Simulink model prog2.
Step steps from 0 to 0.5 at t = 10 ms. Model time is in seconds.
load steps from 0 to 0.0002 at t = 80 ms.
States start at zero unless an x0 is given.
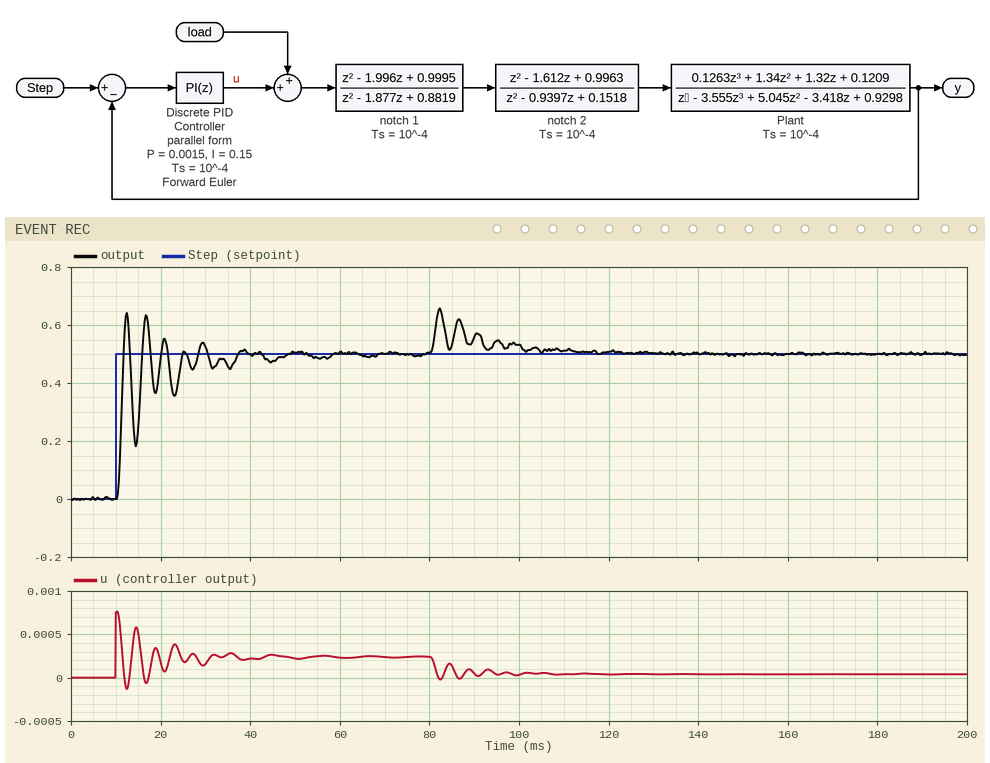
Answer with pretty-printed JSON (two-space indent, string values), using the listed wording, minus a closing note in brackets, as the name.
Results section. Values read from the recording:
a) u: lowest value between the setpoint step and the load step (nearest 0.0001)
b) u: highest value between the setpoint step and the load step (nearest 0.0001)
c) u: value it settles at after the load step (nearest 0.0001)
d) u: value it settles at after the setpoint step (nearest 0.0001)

{
  "u: lowest value between the setpoint step and the load step": "-0.0001",
  "u: highest value between the setpoint step and the load step": "0.0008",
  "u: value it settles at after the load step": "0.0000",
  "u: value it settles at after the setpoint step": "0.0002"
}
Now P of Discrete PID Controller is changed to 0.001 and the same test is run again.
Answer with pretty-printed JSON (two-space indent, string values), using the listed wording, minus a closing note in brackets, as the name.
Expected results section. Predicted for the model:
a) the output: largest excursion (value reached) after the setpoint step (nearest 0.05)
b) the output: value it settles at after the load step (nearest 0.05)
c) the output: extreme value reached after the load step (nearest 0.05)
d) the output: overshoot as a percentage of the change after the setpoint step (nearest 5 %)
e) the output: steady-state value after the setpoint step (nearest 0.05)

{
  "the output: largest excursion (value reached) after the setpoint step": "0.55",
  "the output: value it settles at after the load step": "0.50",
  "the output: extreme value reached after the load step": "0.70",
  "the output: overshoot as a percentage of the change after the setpoint step": "15 %",
  "the output: steady-state value after the setpoint step": "0.50"
}
